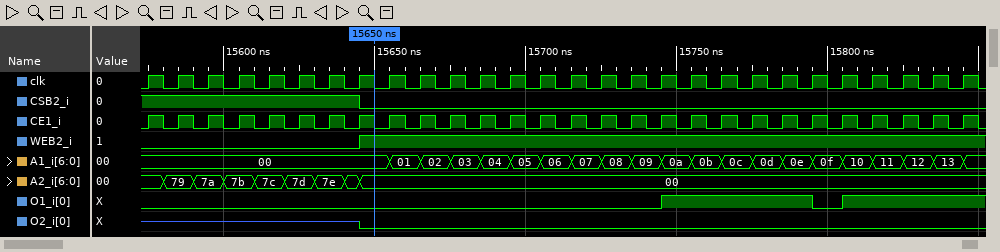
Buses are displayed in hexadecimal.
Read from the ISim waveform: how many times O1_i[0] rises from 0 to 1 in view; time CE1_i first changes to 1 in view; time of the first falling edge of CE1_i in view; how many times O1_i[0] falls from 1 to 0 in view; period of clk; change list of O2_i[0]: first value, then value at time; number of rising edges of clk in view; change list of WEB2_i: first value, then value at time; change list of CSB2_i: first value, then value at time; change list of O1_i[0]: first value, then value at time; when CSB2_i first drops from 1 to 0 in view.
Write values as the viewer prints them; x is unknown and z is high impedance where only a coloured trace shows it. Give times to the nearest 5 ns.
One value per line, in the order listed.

2
15575 ns
15580 ns
1
10 ns
z, 0 at 15645 ns
28
0, 1 at 15645 ns
1, 0 at 15645 ns
0, 1 at 15745 ns, 0 at 15795 ns, 1 at 15805 ns
15645 ns
